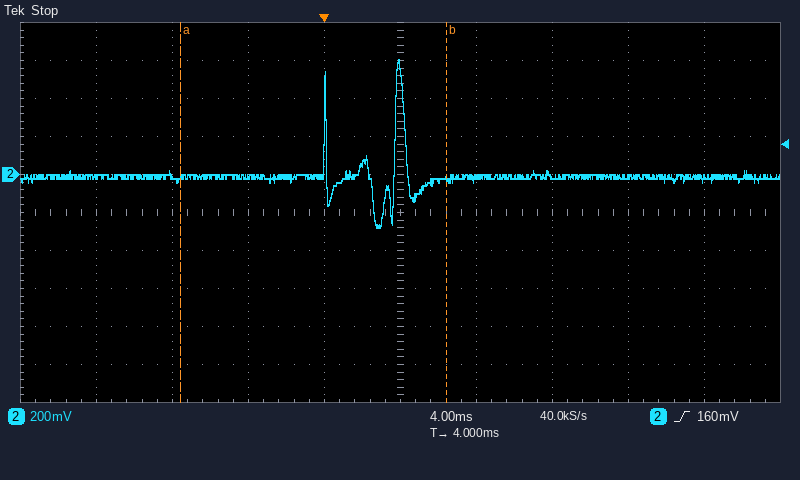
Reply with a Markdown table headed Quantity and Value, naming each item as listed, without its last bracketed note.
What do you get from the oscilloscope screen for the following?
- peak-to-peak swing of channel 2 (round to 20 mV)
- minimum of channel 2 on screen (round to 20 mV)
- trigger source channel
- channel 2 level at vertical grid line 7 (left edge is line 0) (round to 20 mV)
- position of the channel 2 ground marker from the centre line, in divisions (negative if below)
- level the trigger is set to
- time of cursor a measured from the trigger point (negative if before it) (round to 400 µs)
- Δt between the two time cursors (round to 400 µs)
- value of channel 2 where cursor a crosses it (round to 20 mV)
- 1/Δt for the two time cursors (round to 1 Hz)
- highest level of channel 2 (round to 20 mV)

| Quantity | Value |
|---|---|
| peak-to-peak swing of channel 2 | 880 mV |
| minimum of channel 2 on screen | -280 mV |
| trigger source channel | channel 2 |
| channel 2 level at vertical grid line 7 (left edge is line 0) | 0 mV |
| position of the channel 2 ground marker from the centre line, in divisions | +1.0 div |
| level the trigger is set to | 160 mV |
| time of cursor a measured from the trigger point (negative if before it) | -7.6 ms |
| Δt between the two time cursors | 14.0 ms |
| value of channel 2 where cursor a crosses it | -20 mV |
| 1/Δt for the two time cursors | 71 Hz |
| highest level of channel 2 | 600 mV |
